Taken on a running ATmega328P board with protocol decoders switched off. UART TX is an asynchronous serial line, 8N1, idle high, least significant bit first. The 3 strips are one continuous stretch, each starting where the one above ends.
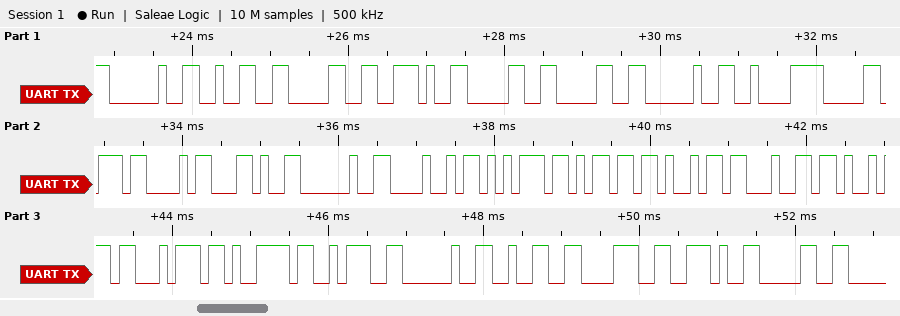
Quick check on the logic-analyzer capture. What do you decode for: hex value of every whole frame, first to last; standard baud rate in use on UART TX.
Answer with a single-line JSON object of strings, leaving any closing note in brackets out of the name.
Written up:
{"hex value of every whole frame, first to last": "0x20 0x32 0x30 0x2E 0x30 0x30 0x20 0xC2 0xB0 0x43 0x2C 0x20 0x48 0x75 0x6D 0x69 0x64 0x69 0x74 0x79 0x3A 0x20 0x32 0x38 0x2E 0x30", "standard baud rate in use on UART TX": "9600 baud"}
